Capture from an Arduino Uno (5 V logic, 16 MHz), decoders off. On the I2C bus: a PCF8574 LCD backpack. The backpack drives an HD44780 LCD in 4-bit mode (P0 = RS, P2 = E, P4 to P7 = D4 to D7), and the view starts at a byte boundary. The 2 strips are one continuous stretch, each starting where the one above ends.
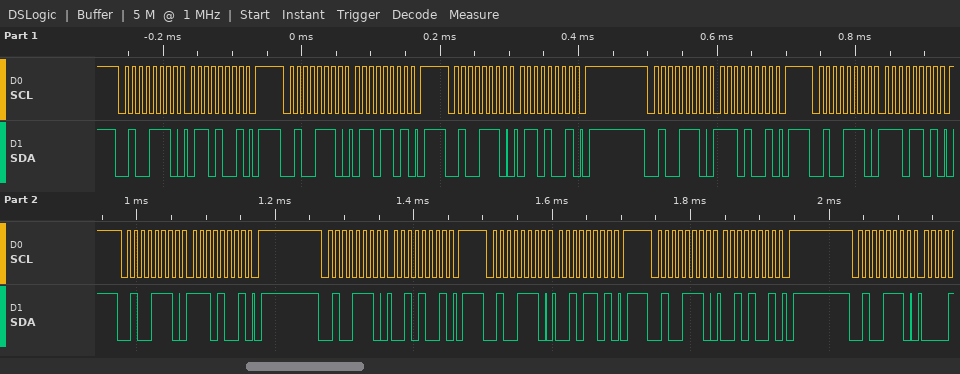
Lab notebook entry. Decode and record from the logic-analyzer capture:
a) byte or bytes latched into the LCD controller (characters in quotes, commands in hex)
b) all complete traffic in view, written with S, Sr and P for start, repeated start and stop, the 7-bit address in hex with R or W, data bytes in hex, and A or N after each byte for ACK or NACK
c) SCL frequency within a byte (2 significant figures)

'n'
S 27W A 69 A P S 27W A 6D A P S 27W A 69 A P S 27W A E9 A P S 27W A ED A P S 27W A E9 A P S 27W A 29 A P S 27W A 2D A P S 27W A 29 A P S 27W A
100 kHz
